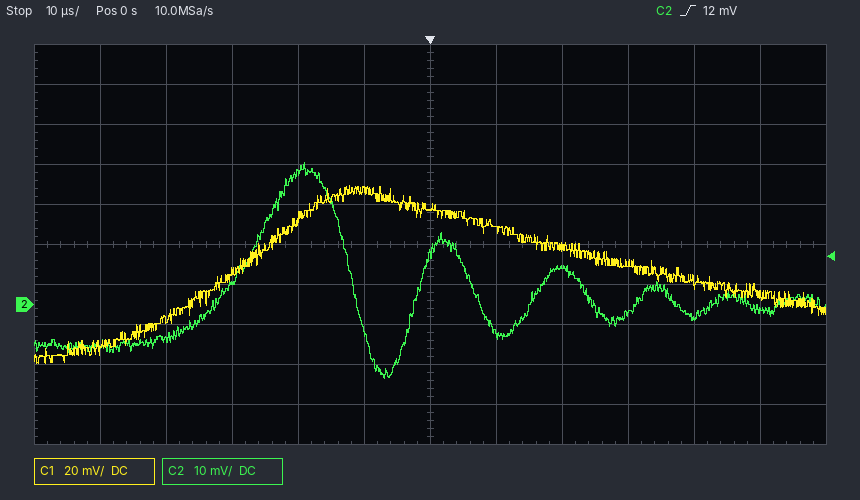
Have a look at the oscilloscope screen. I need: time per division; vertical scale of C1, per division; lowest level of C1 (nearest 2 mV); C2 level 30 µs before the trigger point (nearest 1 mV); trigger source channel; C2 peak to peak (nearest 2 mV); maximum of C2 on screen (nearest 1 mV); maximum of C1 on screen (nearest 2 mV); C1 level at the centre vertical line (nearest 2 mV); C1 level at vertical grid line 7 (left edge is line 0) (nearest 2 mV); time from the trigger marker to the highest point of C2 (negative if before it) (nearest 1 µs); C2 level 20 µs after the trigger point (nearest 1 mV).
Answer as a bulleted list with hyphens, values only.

- 10 µs
- 20 mV
- -30 mV
- 5 mV
- C2
- 54 mV
- 35 mV
- 60 mV
- 48 mV
- 38 mV
- -19 µs
- 9 mV
